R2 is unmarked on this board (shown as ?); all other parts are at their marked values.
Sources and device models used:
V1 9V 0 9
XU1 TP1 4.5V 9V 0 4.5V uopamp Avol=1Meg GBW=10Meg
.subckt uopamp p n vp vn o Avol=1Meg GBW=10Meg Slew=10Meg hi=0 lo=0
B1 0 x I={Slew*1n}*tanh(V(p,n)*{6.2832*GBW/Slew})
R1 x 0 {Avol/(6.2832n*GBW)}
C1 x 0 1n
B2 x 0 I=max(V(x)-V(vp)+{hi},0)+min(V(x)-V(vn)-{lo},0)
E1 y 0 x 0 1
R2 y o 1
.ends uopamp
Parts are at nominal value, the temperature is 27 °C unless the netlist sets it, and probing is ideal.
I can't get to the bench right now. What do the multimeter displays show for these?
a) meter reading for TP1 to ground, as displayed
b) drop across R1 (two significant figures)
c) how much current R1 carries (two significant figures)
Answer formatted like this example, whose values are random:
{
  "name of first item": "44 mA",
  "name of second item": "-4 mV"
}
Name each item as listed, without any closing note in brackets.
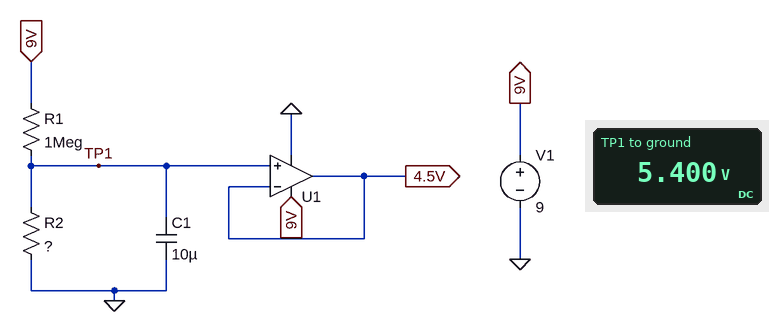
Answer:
{
  "meter reading for TP1 to ground, as displayed": "5.400 V",
  "drop across R1": "3.6 V",
  "how much current R1 carries": "3.6 µA"
}
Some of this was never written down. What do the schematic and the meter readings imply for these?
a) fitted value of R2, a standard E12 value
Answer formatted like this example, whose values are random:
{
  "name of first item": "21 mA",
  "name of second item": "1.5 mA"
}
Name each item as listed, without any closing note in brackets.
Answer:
{
  "fitted value of R2, a standard E12 value": "1.5 MΩ"
}
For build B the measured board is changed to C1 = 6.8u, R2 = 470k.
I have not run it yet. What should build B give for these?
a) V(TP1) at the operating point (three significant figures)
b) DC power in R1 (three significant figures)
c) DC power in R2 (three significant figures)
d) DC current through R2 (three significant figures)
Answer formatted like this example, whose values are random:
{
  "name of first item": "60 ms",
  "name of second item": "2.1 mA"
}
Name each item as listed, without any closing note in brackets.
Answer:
{
  "V(TP1) at the operating point": "2.88 V",
  "DC power in R1": "37.5 µW",
  "DC power in R2": "17.6 µW",
  "DC current through R2": "6.12 µA"
}
